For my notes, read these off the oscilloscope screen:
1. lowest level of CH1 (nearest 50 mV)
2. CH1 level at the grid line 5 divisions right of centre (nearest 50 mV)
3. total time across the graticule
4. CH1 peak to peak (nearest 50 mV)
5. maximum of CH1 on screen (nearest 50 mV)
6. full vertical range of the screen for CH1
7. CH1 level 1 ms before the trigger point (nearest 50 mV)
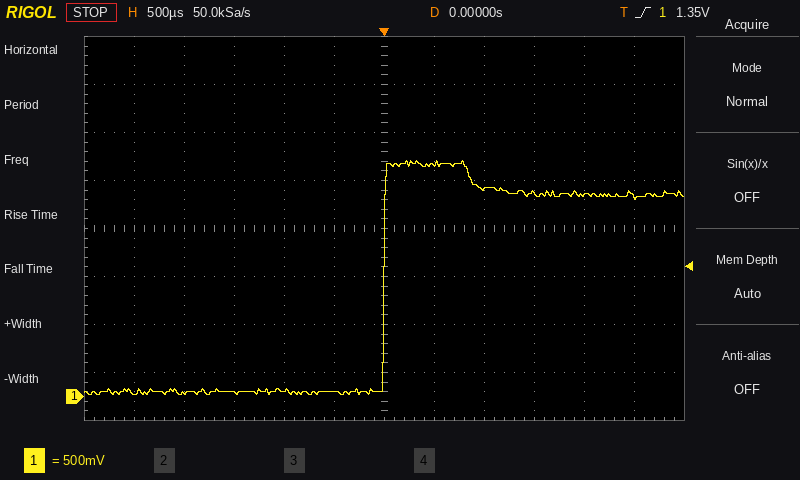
0 mV
2.10 V
6 ms
2.45 V
2.45 V
4 V
50 mV
